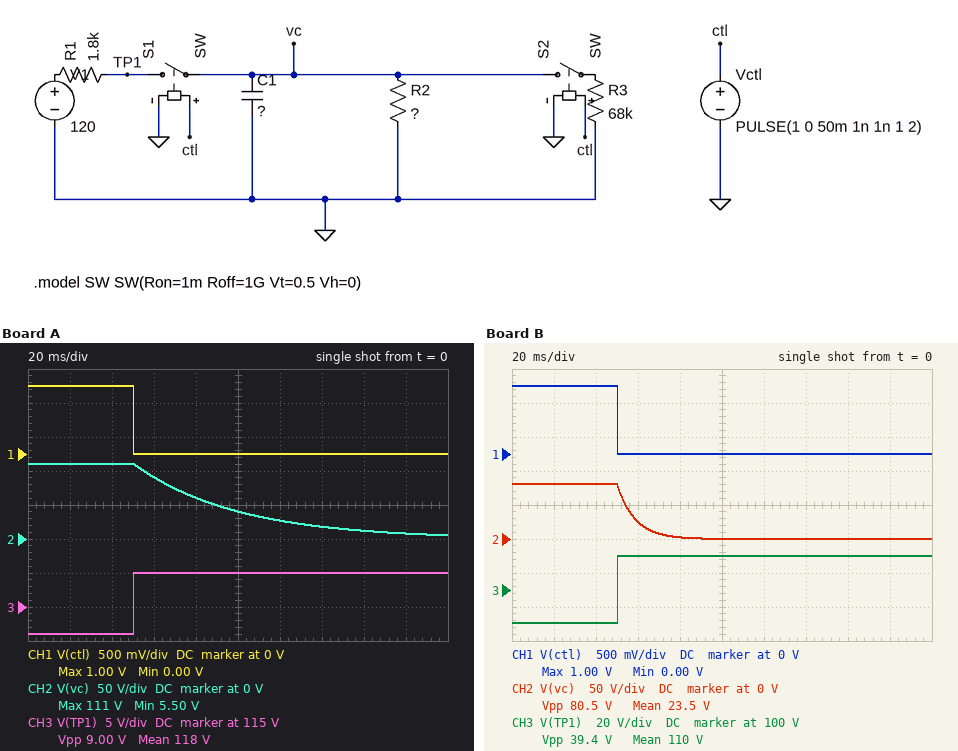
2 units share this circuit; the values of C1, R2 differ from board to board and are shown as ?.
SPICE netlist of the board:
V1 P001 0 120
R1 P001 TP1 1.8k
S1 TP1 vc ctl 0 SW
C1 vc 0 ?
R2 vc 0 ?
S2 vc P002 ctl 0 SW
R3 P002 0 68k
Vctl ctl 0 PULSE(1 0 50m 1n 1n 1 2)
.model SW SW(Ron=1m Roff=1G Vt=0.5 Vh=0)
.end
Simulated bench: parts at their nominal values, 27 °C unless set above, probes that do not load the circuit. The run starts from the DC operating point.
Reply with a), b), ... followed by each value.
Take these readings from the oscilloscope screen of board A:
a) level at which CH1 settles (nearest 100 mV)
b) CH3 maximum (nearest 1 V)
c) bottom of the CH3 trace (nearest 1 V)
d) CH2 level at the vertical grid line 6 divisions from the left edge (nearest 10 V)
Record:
a) 0 V
b) 120 V
c) 111 V
d) 30 V
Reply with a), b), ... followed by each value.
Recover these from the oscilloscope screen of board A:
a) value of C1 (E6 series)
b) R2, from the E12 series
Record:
a) 1.5 µF
b) 33 kΩ
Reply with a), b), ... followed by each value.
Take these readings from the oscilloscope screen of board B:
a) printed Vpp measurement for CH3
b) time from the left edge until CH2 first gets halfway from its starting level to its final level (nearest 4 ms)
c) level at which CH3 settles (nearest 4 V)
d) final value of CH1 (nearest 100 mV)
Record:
a) 39.4 V
b) 56 ms
c) 120 V
d) 0 V
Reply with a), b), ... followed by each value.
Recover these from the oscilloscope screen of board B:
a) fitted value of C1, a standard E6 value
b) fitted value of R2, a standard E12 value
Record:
a) 2.2 µF
b) 3.9 kΩ
